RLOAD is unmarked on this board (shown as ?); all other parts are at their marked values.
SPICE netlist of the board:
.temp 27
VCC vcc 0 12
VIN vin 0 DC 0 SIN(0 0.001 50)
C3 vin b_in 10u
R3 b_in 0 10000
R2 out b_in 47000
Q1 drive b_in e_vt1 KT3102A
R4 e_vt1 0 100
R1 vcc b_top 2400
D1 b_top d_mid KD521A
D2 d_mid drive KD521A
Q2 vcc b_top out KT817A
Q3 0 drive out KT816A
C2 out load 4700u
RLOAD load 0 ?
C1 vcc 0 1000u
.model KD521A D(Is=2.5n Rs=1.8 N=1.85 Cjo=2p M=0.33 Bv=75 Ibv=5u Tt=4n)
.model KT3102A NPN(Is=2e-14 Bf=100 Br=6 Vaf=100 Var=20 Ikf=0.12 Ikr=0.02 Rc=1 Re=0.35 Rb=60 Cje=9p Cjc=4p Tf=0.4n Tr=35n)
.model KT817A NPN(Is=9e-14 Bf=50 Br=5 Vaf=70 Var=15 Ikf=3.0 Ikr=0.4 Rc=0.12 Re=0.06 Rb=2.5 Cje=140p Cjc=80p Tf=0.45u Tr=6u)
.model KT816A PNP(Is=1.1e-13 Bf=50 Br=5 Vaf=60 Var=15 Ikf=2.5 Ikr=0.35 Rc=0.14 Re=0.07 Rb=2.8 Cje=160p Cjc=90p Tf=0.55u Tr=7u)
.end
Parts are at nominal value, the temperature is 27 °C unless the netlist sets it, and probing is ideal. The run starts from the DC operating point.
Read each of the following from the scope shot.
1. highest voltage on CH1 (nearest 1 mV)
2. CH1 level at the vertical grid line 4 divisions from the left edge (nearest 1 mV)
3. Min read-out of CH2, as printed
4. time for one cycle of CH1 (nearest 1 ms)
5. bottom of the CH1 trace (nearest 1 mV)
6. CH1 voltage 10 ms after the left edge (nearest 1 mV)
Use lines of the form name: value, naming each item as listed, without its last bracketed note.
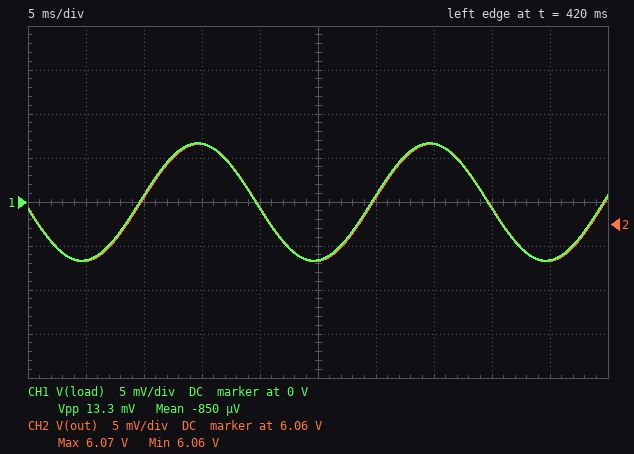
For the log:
highest voltage on CH1: 7 mV
CH1 level at the vertical grid line 4 divisions from the left edge: -1 mV
Min read-out of CH2, as printed: 6.06 V
time for one cycle of CH1: 20 ms
bottom of the CH1 trace: -7 mV
CH1 voltage 10 ms after the left edge: 1 mV
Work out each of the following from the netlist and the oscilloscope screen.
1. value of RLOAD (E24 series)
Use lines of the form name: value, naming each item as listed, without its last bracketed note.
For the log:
value of RLOAD: 22 Ω
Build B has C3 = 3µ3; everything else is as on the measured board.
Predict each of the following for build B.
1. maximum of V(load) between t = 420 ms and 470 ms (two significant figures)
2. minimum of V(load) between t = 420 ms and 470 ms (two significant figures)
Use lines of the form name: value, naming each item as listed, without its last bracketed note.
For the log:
maximum of V(load) between t = 420 ms and 470 ms: 6.4 mV
minimum of V(load) between t = 420 ms and 470 ms: -6.4 mV
